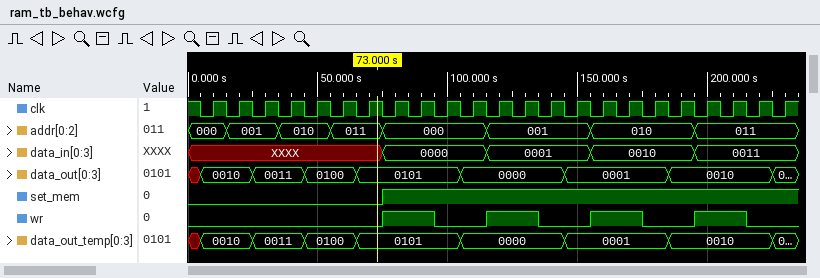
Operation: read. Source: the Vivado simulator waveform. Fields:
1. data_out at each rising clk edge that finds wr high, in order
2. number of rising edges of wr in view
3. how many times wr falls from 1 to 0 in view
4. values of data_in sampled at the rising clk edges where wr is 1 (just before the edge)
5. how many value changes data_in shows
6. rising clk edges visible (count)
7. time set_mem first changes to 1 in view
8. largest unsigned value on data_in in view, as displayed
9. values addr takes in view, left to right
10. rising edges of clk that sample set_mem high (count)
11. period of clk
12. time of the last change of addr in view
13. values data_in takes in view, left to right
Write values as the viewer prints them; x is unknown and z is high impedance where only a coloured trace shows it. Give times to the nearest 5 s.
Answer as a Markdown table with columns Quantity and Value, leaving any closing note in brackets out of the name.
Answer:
| Quantity | Value |
|---|---|
| data_out at each rising clk edge that finds wr high, in order | 0101, 0101, 0000, 0000, 0001, 0001, 0010, 0010 |
| number of rising edges of wr in view | 4 |
| how many times wr falls from 1 to 0 in view | 4 |
| values of data_in sampled at the rising clk edges where wr is 1 | 0000, 0000, 0001, 0001, 0010, 0010, 0011, 0011 |
| how many value changes data_in shows | 4 |
| rising clk edges visible | 23 |
| time set_mem first changes to 1 in view | 75 s |
| largest unsigned value on data_in in view, as displayed | 0011 |
| values addr takes in view, left to right | 000, 001, 010, 011, 000, 001, 010, 011 |
| rising edges of clk that sample set_mem high | 16 |
| period of clk | 10 s |
| time of the last change of addr in view | 195 s |
| values data_in takes in view, left to right | XXXX, 0000, 0001, 0010, 0011 |
